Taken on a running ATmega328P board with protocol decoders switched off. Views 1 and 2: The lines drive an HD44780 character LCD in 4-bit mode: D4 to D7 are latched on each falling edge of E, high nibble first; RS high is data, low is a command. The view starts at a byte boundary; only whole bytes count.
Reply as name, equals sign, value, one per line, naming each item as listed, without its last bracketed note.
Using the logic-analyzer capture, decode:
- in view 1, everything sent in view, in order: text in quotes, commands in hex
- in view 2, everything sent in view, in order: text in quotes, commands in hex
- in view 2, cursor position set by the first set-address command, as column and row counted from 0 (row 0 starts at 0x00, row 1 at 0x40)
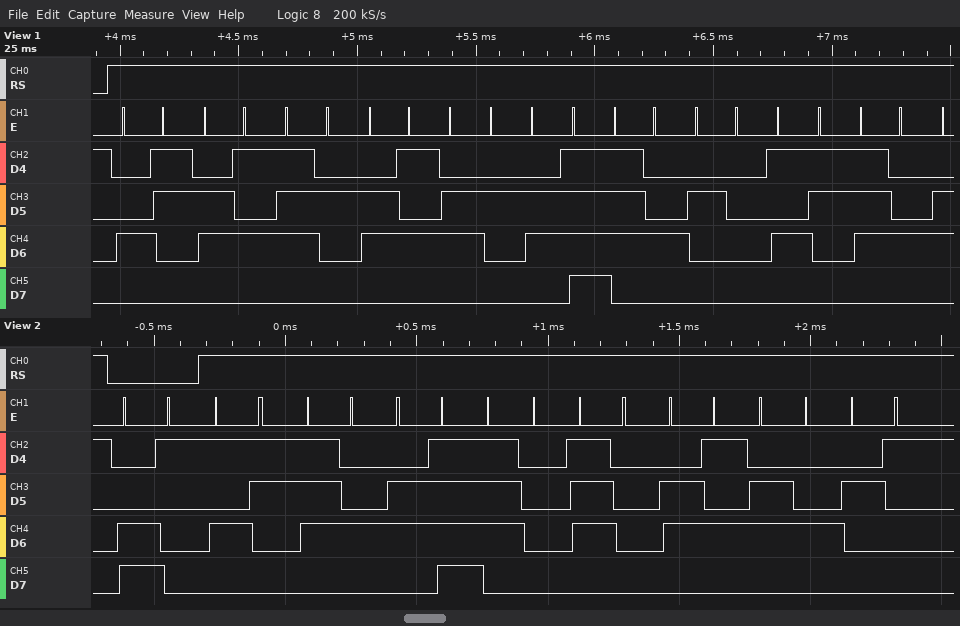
in view 1, everything sent in view, in order: text in quotes, commands in hex = "Cerebot St"
in view 2, everything sent in view, in order: text in quotes, commands in hex = 0xC1 "Stopped!"
in view 2, cursor position set by the first set-address command, as column and row counted from 0 = column 1, row 1
